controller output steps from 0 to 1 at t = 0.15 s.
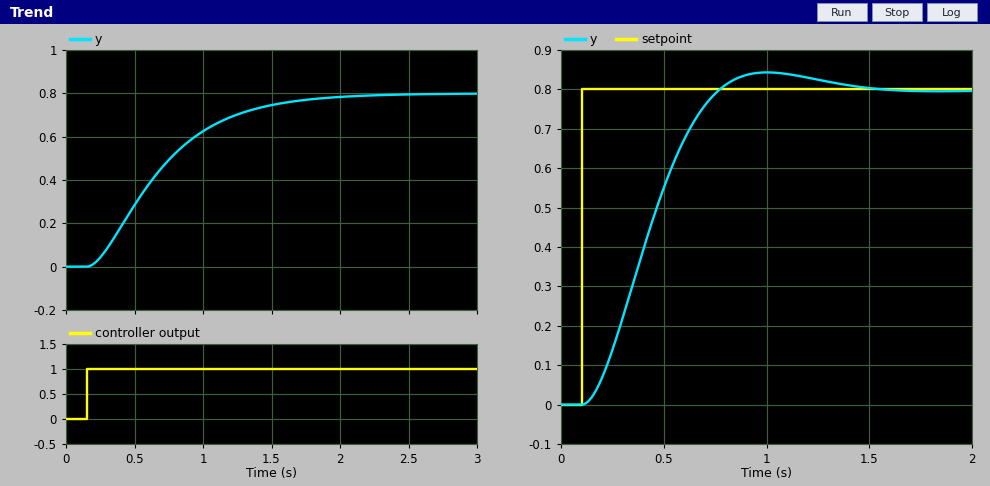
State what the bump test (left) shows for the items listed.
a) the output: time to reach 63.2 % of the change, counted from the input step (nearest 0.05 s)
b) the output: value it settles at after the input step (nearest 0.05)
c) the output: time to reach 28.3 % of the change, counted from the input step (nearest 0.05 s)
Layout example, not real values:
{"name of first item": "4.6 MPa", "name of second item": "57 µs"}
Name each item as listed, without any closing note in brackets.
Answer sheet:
{"the output: time to reach 63.2 % of the change, counted from the input step": "0.60 s", "the output: value it settles at after the input step": "0.80", "the output: time to reach 28.3 % of the change, counted from the input step": "0.30 s"}
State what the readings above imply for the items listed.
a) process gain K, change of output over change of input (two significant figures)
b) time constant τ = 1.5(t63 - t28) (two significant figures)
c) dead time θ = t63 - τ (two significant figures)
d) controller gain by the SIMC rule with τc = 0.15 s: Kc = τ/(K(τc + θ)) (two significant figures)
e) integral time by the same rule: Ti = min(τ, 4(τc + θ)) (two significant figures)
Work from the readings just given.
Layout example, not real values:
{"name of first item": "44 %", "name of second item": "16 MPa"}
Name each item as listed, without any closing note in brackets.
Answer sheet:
{"process gain K, change of output over change of input": "0.80", "time constant τ = 1.5(t63 - t28)": "0.45 s", "dead time θ = t63 - τ": "0.15 s", "controller gain by the SIMC rule with τc = 0.15 s: Kc = τ/(K(τc + θ))": "1.9", "integral time by the same rule: Ti = min(τ, 4(τc + θ))": "0.45 s"}
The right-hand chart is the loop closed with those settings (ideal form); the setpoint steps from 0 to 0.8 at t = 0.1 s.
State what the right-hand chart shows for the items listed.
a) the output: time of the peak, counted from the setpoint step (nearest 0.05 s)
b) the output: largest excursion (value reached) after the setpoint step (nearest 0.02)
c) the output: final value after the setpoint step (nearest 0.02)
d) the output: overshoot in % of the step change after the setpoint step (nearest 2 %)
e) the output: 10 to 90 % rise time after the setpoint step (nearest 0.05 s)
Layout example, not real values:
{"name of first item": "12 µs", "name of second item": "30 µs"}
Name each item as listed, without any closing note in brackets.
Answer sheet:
{"the output: time of the peak, counted from the setpoint step": "0.90 s", "the output: largest excursion (value reached) after the setpoint step": "0.84", "the output: final value after the setpoint step": "0.80", "the output: overshoot in % of the step change after the setpoint step": "6 %", "the output: 10 to 90 % rise time after the setpoint step": "0.45 s"}
